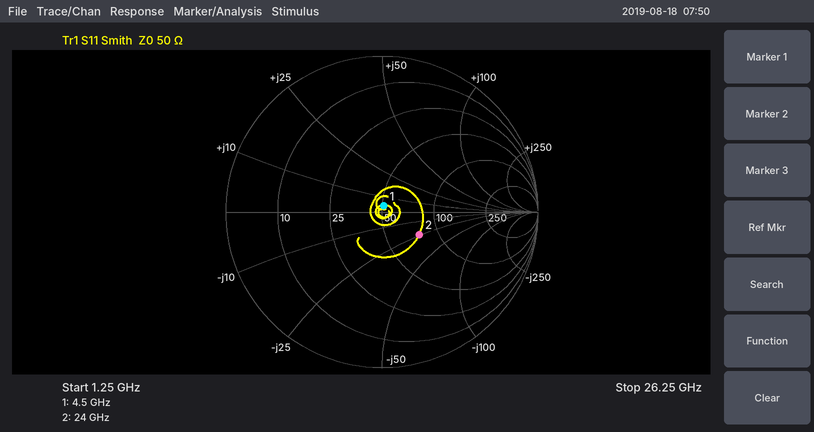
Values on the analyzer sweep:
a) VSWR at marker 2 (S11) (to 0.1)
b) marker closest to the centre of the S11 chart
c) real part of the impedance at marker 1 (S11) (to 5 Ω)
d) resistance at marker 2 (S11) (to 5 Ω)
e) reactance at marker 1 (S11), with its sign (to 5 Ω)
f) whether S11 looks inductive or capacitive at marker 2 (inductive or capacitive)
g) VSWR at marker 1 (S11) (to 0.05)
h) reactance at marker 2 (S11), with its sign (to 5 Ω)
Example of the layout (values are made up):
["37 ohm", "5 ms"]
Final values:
["1.8", "marker 1", "50 Ω", "75 Ω", "+5 Ω", "capacitive", "1.10", "-25 Ω"]
